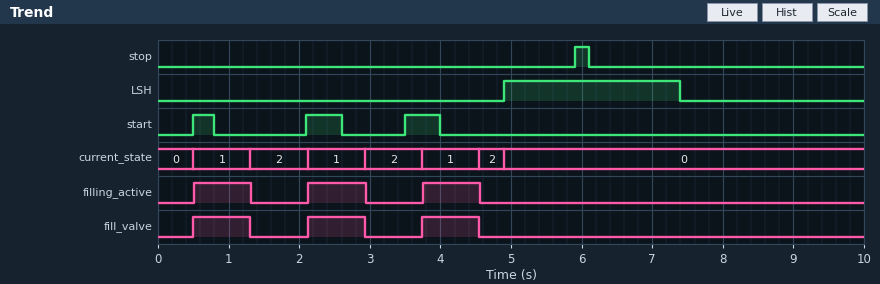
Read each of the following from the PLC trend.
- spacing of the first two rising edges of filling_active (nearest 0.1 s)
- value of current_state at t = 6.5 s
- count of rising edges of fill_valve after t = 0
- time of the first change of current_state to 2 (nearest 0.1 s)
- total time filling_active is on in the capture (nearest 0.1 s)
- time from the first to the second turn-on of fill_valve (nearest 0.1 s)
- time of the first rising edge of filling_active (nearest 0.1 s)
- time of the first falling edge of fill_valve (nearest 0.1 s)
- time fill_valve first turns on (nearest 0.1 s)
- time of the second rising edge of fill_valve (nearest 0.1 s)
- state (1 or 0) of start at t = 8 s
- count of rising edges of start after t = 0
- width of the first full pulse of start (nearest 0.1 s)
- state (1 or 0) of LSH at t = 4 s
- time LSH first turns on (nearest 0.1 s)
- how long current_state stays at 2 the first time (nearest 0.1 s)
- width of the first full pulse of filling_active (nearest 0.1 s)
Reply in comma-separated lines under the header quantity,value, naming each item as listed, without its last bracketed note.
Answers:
quantity,value
spacing of the first two rising edges of filling_active,1.6 s
value of current_state at t = 6.5 s,0
count of rising edges of fill_valve after t = 0,3
time of the first change of current_state to 2,1.3 s
total time filling_active is on in the capture,2.4 s
time from the first to the second turn-on of fill_valve,1.6 s
time of the first rising edge of filling_active,0.5 s
time of the first falling edge of fill_valve,1.3 s
time fill_valve first turns on,0.5 s
time of the second rising edge of fill_valve,2.1 s
state (1 or 0) of start at t = 8 s,0
count of rising edges of start after t = 0,3
width of the first full pulse of start,0.3 s
state (1 or 0) of LSH at t = 4 s,0
time LSH first turns on,4.9 s
how long current_state stays at 2 the first time,0.8 s
width of the first full pulse of filling_active,0.8 s
